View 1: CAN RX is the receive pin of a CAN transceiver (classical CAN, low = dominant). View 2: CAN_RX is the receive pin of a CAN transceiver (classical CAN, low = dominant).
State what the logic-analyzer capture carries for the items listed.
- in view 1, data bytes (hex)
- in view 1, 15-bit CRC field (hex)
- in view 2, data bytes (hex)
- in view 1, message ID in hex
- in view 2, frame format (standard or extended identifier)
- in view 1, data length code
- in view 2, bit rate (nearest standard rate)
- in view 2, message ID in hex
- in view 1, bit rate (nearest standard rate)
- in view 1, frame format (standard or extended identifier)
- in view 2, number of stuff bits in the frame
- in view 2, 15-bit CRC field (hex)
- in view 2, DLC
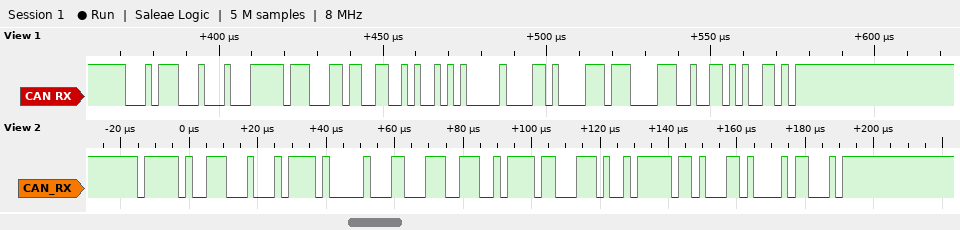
FF 1B 32 95 00 68 77 0E
0x26A6
BD 00 C7 39 7B 1D 2F E8
0x171
standard
8
500 kbit/s
0x7E7
500 kbit/s
standard
3
0x6858
8
